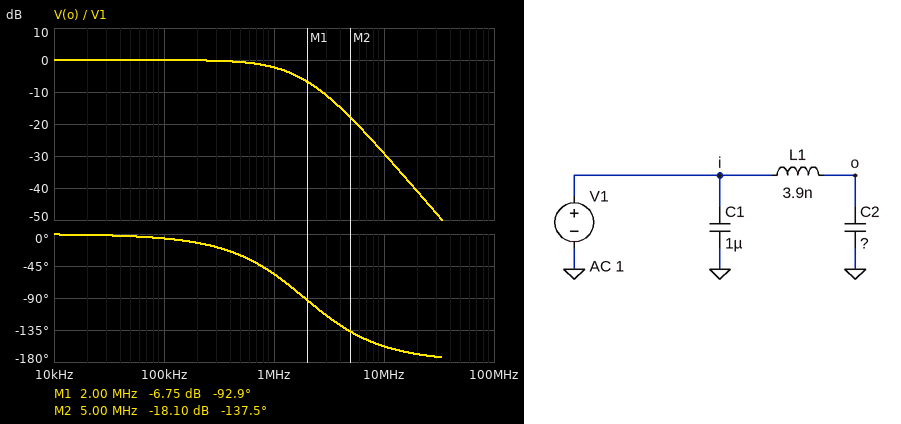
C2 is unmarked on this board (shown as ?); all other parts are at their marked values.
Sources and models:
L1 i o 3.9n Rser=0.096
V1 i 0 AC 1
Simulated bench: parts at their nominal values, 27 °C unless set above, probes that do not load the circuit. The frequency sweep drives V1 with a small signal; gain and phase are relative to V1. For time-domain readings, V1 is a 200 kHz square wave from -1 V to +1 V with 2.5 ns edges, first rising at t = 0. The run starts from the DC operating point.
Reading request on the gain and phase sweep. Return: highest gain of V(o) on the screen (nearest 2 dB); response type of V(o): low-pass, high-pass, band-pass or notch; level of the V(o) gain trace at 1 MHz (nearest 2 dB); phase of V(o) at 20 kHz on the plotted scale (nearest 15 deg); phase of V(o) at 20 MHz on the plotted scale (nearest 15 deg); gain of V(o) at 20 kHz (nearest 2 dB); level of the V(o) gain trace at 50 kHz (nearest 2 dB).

0 dB
low-pass
-2 dB
0 deg
-165 deg
0 dB
0 dB
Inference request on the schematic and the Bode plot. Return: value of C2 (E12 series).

1.8 µF
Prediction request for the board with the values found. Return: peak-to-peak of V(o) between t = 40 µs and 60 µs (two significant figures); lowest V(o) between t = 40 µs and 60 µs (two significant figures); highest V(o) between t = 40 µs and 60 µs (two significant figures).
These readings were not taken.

2.0 V
-1.0 V
1.0 V
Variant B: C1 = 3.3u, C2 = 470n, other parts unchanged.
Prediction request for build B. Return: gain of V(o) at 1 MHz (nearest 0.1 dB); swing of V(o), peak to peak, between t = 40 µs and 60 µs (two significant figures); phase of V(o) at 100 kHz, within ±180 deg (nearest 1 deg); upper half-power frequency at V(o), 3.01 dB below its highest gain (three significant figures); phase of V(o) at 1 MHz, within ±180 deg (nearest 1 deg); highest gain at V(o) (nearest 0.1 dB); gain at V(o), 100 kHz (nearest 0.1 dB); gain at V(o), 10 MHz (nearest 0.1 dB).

0.3 dB
2.6 V
-2 deg
4.30 MHz
-17 deg
1.0 dB
0 dB
-16.7 dB
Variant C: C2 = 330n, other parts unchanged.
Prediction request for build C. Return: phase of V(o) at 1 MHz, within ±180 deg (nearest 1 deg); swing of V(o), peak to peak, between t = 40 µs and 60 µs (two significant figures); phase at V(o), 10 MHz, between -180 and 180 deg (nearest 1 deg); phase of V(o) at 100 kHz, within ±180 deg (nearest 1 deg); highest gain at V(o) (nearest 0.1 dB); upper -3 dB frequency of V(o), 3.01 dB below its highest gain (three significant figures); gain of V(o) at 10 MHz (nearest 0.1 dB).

-12 deg
2.9 V
-154 deg
-1 deg
2.0 dB
5.25 MHz
-13.1 dB
